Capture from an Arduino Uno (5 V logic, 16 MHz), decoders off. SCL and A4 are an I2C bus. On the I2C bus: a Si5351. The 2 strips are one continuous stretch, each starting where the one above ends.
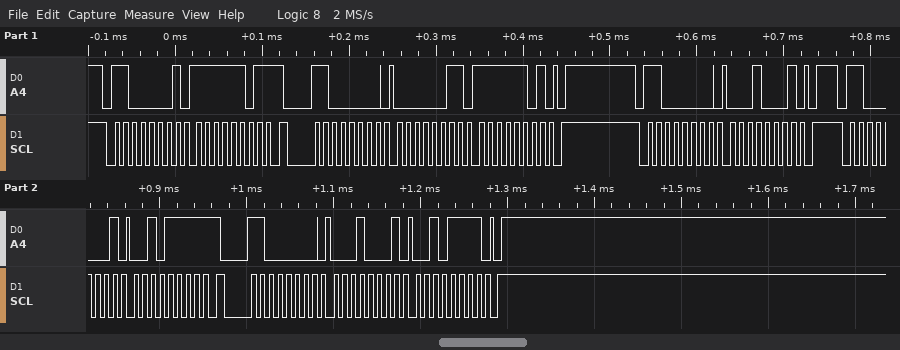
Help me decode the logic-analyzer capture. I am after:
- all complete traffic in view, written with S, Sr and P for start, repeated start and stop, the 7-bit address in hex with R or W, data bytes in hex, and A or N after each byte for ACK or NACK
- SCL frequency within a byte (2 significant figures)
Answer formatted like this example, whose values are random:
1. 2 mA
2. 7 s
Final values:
1. S 60R A FD N Sr 60W A 03 A FD A P S 60W A 11 A P S 60R A 2F N Sr 60W A 11 A 2F A P
2. 100 kHz
